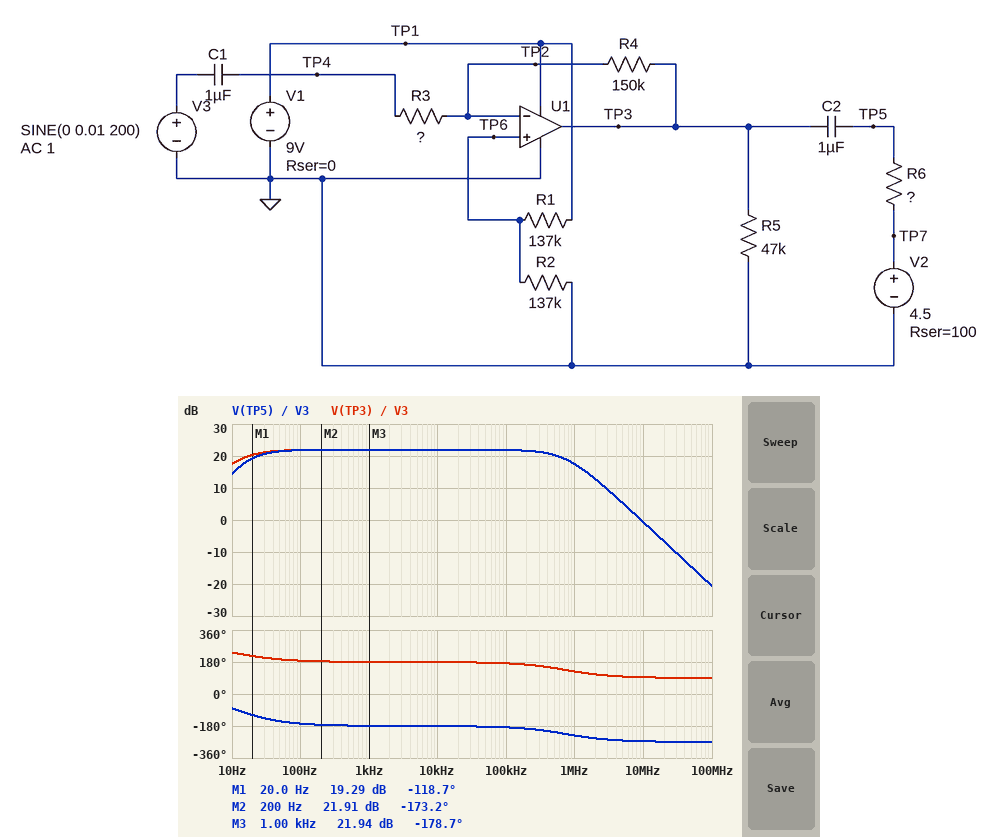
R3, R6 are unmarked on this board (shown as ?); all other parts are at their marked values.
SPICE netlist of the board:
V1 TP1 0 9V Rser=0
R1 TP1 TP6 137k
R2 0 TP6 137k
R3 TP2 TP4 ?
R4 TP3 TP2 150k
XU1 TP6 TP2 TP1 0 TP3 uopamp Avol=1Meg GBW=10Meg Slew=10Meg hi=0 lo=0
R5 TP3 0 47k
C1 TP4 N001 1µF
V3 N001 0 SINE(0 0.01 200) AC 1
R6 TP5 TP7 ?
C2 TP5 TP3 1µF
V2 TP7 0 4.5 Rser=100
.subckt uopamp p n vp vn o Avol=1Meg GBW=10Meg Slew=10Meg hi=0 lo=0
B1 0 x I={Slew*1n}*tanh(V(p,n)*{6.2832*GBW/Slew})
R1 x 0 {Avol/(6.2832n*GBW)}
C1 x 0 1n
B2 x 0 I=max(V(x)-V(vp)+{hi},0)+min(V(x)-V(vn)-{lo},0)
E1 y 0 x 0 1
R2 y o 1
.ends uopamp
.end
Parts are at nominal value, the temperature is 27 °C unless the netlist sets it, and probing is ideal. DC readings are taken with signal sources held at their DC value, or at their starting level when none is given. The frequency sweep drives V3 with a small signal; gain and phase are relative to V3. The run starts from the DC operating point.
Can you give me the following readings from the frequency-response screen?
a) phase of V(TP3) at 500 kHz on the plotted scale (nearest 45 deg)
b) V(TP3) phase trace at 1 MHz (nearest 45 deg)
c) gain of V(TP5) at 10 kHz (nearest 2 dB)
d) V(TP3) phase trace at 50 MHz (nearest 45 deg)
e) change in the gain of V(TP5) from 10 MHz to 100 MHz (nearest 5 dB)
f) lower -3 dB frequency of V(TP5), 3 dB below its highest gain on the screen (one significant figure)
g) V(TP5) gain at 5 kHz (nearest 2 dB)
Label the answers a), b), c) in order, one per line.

a) 135 deg
b) 135 deg
c) 22 dB
d) 90 deg
e) -20 dB
f) 20 Hz
g) 22 dB
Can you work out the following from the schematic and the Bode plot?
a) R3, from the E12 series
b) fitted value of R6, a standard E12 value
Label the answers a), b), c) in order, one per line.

a) 12 kΩ
b) 15 kΩ
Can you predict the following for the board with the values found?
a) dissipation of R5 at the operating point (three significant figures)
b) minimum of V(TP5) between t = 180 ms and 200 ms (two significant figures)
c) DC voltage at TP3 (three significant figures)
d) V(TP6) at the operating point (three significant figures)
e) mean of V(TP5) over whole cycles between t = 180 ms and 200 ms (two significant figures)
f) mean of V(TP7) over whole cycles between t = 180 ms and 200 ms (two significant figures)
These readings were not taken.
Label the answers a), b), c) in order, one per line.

a) 431 µW
b) 4.4 V
c) 4.50 V
d) 4.50 V
e) 4.5 V
f) 4.5 V
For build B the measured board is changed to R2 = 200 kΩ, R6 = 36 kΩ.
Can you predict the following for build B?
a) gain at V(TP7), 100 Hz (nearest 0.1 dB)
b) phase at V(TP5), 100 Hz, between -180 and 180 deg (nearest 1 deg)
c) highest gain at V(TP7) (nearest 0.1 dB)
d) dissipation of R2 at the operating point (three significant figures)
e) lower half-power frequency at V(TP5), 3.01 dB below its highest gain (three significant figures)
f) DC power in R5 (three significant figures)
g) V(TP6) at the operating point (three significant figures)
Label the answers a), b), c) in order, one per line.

a) -29.3 dB
b) -170 deg
c) -29.2 dB
d) 143 µW
e) 14.5 Hz
f) 607 µW
g) 5.34 V
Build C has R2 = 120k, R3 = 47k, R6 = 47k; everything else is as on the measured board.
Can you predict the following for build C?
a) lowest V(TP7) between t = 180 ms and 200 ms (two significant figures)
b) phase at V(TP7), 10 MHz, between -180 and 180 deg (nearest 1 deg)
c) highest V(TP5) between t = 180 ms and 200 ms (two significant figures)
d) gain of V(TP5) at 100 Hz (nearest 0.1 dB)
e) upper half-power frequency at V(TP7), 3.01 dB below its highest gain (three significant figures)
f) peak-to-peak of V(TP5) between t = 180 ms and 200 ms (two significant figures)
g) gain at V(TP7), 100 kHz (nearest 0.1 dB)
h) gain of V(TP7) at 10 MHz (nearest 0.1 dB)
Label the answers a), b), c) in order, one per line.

a) 4.5 V
b) 103 deg
c) 4.5 V
d) 10.1 dB
e) 2.39 MHz
f) 64 mV
g) -43.4 dB
h) -56.1 dB
